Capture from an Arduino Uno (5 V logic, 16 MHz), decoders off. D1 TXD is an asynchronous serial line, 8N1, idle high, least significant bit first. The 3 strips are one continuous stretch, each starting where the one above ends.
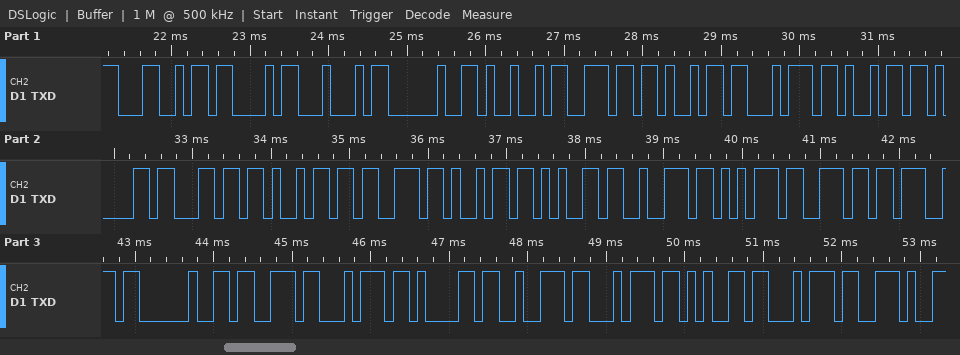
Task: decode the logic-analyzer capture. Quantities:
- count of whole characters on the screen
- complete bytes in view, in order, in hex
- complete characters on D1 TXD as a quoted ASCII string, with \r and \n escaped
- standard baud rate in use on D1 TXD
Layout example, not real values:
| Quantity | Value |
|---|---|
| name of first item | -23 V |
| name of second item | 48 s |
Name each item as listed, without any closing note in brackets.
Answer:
| Quantity | Value |
|---|---|
| count of whole characters on the screen | 28 |
| complete bytes in view, in order, in hex | 4C 43 44 20 49 6E 69 74 69 61 6C 69 73 69 65 72 75 6E 67 20 73 74 61 72 74 65 74 2E |
| complete characters on D1 TXD as a quoted ASCII string, with \r and \n escaped | "LCD Initialisierung startet." |
| standard baud rate in use on D1 TXD | 9600 baud |
